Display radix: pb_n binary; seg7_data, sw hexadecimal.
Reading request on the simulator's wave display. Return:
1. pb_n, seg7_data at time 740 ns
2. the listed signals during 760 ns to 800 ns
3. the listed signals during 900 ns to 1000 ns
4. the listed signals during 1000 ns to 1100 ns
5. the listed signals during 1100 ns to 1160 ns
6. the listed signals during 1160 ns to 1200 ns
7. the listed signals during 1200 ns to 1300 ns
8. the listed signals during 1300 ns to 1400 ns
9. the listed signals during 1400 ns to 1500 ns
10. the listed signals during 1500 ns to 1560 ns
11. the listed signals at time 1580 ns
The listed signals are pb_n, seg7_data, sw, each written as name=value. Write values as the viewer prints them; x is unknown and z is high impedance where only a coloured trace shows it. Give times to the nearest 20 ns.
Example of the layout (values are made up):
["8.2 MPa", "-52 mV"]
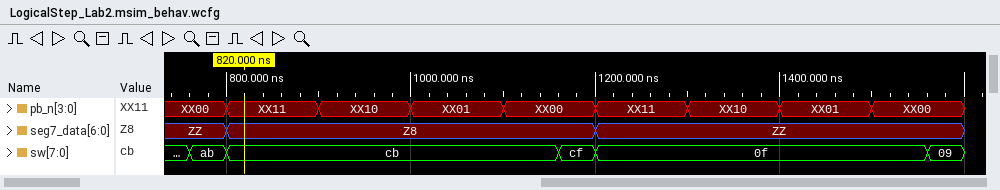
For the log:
["pb_n=XX00, seg7_data=ZZ", "pb_n=XX00, seg7_data=ZZ, sw=ab", "pb_n=XX10, seg7_data=Z8, sw=cb", "pb_n=XX01, seg7_data=Z8, sw=cb", "pb_n=XX00, seg7_data=Z8, sw=cb", "pb_n=XX00, seg7_data=Z8, sw=cf", "pb_n=XX11, seg7_data=ZZ, sw=0f", "pb_n=XX10, seg7_data=ZZ, sw=0f", "pb_n=XX01, seg7_data=ZZ, sw=0f", "pb_n=XX00, seg7_data=ZZ, sw=0f", "pb_n=XX00, seg7_data=ZZ, sw=09"]
